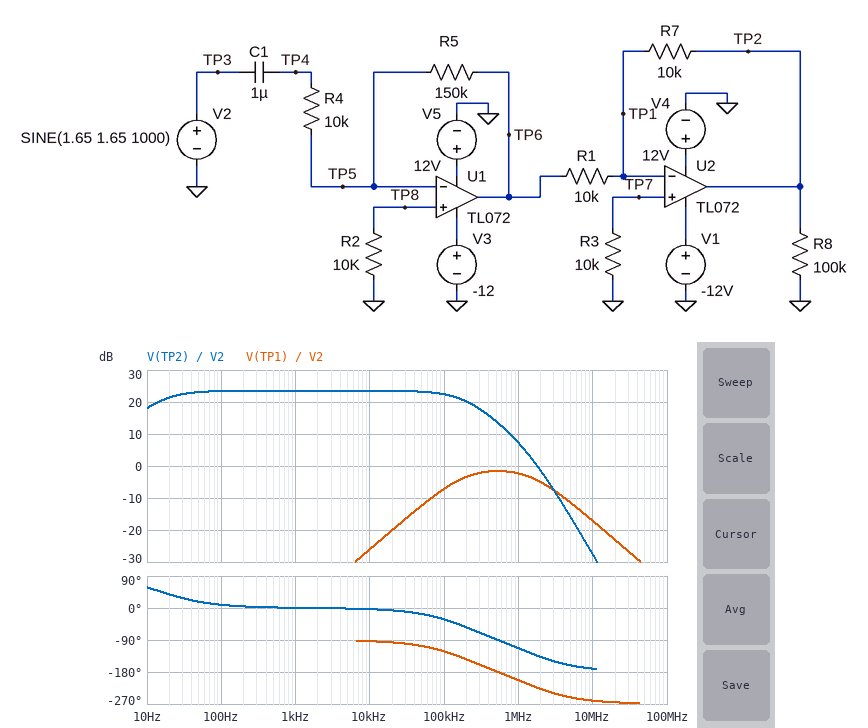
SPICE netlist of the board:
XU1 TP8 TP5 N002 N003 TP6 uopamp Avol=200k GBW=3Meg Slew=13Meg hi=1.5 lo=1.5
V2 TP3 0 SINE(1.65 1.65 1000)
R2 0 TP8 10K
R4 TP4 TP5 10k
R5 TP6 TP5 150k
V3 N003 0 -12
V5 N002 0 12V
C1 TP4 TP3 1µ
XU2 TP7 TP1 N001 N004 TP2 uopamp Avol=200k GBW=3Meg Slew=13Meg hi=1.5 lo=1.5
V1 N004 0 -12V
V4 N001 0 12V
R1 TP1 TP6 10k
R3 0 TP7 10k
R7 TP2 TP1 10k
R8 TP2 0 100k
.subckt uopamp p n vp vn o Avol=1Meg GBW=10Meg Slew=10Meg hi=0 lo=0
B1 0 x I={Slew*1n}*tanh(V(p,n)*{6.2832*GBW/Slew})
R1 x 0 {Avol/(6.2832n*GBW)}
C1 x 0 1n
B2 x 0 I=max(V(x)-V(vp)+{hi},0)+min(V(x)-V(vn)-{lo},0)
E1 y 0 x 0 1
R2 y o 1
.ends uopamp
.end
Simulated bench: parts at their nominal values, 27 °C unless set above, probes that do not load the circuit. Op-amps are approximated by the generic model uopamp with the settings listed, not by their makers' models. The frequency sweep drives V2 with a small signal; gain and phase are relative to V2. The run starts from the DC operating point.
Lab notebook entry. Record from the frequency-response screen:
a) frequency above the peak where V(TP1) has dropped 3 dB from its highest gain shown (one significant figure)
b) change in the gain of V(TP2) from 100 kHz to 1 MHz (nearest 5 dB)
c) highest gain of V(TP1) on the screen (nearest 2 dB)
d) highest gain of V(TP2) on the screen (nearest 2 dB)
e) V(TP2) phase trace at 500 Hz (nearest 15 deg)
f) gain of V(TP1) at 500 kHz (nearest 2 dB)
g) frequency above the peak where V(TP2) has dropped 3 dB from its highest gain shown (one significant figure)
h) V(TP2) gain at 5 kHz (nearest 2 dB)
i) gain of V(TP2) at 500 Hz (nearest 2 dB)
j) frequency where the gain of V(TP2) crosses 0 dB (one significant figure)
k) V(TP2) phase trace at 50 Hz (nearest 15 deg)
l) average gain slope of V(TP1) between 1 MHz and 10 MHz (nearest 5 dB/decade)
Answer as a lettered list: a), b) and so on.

a) 2 MHz
b) -15 dB
c) -2 dB
d) 24 dB
e) 0 deg
f) -2 dB
g) 200 kHz
h) 24 dB
i) 24 dB
j) 2 MHz
k) 15 deg
l) -15 dB/decade
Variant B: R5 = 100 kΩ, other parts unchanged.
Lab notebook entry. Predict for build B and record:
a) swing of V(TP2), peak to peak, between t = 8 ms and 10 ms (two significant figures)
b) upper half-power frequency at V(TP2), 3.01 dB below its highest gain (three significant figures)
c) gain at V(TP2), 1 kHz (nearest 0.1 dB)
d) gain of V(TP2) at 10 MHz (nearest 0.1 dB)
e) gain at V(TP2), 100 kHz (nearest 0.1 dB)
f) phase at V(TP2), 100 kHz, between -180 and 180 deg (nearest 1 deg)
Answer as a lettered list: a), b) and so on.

a) 21 V
b) 264 kHz
c) 20.0 dB
d) -27.9 dB
e) 19.4 dB
f) -24 deg
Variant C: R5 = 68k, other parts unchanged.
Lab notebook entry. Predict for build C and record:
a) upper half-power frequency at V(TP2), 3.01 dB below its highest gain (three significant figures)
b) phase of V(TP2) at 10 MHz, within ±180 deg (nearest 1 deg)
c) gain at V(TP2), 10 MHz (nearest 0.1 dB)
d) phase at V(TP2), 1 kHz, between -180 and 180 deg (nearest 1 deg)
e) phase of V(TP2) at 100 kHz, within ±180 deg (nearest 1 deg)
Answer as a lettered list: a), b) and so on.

a) 363 kHz
b) -169 deg
c) -28.2 dB
d) 1 deg
e) -18 deg
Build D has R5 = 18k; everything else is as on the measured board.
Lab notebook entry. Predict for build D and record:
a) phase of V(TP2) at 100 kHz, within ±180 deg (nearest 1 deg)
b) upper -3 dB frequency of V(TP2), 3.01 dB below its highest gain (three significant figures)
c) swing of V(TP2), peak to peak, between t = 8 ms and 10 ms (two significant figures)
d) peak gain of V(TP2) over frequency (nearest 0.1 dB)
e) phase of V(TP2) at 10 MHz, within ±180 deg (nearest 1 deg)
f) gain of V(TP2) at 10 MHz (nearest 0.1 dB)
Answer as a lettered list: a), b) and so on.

a) -9 deg
b) 800 kHz
c) 5.9 V
d) 5.1 dB
e) -165 deg
f) -30.9 dB
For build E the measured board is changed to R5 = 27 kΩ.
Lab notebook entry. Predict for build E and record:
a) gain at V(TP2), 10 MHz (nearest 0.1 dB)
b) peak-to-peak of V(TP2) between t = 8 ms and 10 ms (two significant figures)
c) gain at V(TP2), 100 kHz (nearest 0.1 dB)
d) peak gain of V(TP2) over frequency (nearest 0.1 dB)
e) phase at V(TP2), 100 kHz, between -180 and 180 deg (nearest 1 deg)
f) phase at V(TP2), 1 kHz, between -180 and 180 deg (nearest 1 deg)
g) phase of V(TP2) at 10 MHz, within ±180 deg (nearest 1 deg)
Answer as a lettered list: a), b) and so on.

a) -29.8 dB
b) 8.9 V
c) 8.5 dB
d) 8.6 dB
e) -11 deg
f) 1 deg
g) -167 deg
